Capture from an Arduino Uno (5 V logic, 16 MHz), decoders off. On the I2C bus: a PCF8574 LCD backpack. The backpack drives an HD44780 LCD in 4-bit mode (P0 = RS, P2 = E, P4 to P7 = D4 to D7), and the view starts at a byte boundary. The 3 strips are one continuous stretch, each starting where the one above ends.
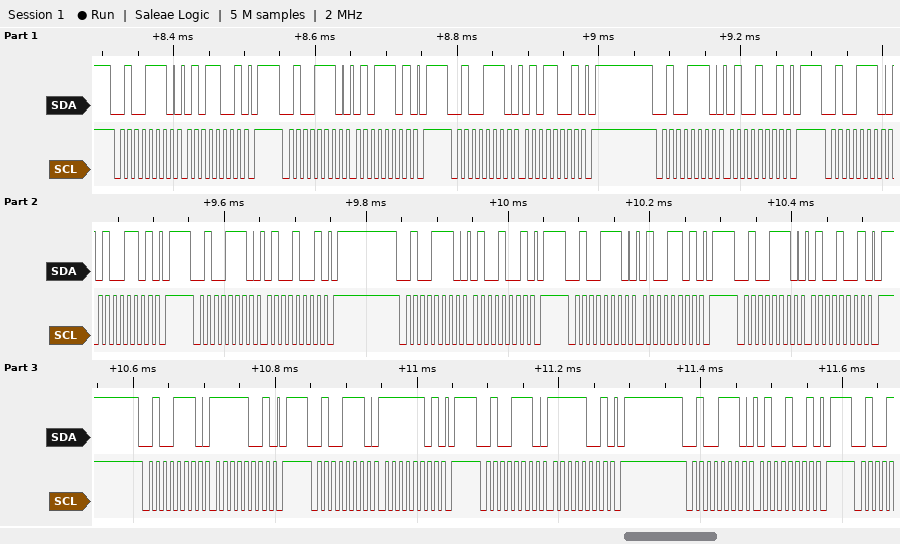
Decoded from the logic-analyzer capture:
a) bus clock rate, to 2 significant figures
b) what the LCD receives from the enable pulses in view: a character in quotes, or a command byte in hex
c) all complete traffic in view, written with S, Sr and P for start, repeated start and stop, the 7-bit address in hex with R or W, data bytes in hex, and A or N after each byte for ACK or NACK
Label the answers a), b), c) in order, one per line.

a) 100 kHz
b) 'T' 'O'
c) S 27W A 59 A P S 27W A 5D A P S 27W A 59 A P S 27W A 49 A P S 27W A 4D A P S 27W A 49 A P S 27W A 49 A P S 27W A 4D A P S 27W A 49 A P S 27W A F9 A P S 27W A FD A P S 27W A F9 A P S 27W A 49 A P
